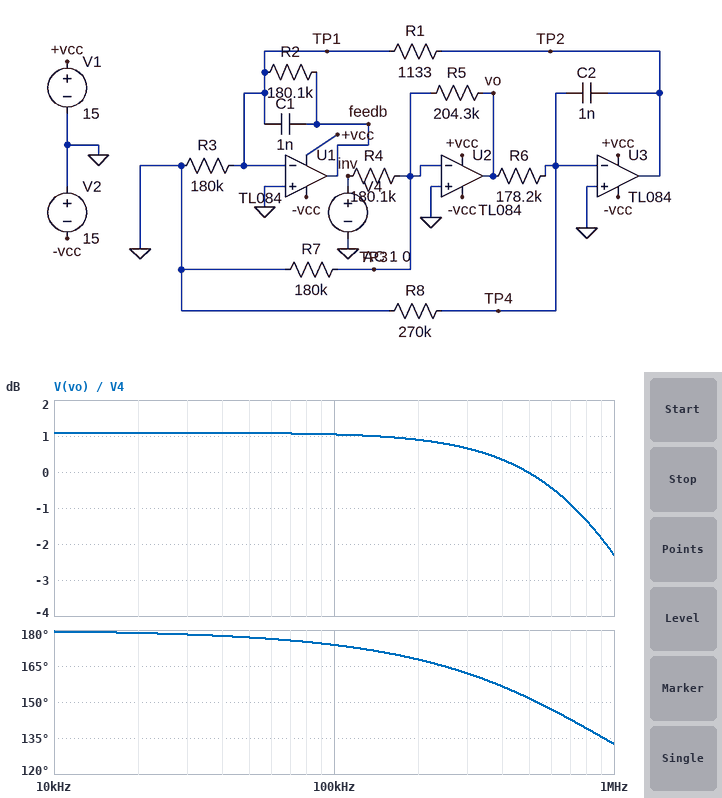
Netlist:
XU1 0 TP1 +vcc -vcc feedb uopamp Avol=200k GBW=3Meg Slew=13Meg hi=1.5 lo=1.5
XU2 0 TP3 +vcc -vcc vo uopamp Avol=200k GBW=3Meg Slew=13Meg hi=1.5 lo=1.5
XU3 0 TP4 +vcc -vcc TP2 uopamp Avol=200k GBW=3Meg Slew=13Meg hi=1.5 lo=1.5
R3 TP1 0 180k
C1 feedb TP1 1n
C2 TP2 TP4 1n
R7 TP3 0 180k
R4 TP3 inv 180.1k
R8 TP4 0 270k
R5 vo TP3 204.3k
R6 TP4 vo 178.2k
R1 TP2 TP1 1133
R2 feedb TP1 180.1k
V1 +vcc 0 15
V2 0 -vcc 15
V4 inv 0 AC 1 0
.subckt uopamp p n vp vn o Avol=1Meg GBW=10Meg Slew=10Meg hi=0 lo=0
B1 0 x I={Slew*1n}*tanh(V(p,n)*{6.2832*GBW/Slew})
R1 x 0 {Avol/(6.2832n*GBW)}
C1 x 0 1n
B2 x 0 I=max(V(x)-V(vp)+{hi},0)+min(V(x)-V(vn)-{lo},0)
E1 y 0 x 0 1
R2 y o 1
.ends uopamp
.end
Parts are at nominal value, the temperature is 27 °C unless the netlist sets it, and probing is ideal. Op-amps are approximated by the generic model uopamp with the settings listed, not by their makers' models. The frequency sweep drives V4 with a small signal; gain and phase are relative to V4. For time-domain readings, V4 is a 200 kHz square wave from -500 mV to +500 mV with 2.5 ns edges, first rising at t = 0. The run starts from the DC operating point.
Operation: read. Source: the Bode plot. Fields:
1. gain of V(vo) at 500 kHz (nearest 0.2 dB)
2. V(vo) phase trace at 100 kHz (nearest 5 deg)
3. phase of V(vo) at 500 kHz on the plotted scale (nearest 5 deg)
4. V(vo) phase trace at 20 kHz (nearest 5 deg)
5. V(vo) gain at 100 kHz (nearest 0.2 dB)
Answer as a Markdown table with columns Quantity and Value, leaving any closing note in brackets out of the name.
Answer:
| Quantity | Value |
|---|---|
| gain of V(vo) at 500 kHz | 0 dB |
| V(vo) phase trace at 100 kHz | 175 deg |
| phase of V(vo) at 500 kHz on the plotted scale | 150 deg |
| V(vo) phase trace at 20 kHz | 180 deg |
| V(vo) gain at 100 kHz | 1.0 dB |
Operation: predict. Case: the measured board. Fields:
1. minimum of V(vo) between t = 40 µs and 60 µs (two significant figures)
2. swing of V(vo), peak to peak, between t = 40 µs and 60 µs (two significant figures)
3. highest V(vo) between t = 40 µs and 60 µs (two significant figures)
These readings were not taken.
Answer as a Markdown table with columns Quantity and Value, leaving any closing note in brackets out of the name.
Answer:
| Quantity | Value |
|---|---|
| minimum of V(vo) between t = 40 µs and 60 µs | -570 mV |
| swing of V(vo), peak to peak, between t = 40 µs and 60 µs | 1.1 V |
| highest V(vo) between t = 40 µs and 60 µs | 570 mV |
